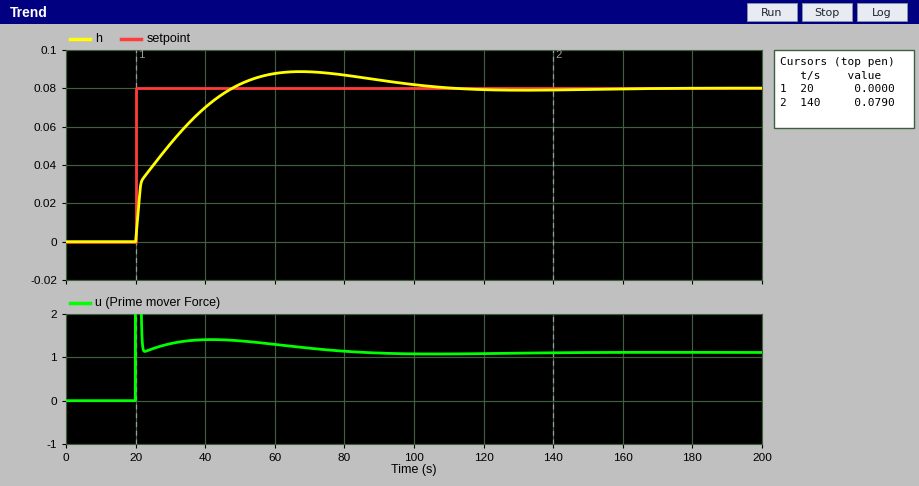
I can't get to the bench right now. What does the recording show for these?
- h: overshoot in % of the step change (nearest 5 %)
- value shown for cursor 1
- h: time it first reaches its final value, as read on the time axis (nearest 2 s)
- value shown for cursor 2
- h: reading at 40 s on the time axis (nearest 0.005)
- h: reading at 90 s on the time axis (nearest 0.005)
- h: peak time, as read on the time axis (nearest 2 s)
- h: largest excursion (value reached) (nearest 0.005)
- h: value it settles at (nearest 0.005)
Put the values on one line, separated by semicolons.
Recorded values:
10 %; 0.0000; 48 s; 0.0790; 0.070; 0.085; 68 s; 0.090; 0.080
